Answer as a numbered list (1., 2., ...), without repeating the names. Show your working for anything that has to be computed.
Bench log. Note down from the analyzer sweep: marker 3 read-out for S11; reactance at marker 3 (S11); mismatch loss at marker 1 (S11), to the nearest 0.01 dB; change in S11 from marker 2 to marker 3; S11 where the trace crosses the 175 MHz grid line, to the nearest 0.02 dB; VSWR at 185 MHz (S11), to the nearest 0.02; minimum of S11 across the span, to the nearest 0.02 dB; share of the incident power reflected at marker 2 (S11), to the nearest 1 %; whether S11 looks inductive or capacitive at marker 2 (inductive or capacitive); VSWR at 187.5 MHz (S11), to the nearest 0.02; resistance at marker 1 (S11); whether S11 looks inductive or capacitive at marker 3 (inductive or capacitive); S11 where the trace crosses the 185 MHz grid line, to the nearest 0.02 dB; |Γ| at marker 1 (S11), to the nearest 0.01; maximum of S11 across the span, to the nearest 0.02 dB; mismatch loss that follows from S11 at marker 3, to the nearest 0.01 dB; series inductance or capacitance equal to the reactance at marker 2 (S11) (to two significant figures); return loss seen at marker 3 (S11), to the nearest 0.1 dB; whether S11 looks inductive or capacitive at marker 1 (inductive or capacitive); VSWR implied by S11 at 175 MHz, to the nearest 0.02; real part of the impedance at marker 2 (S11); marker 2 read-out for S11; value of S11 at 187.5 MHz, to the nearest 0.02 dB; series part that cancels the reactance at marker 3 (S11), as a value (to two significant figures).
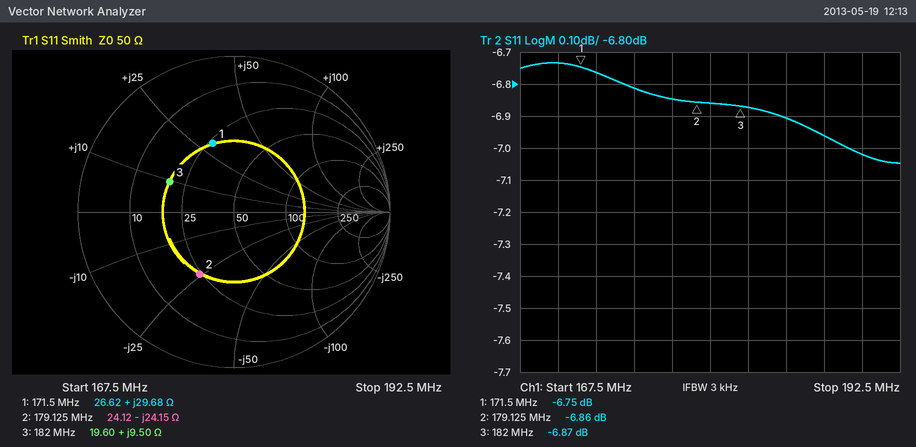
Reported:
1. -6.87 dB
2. +9.50 Ω
3. −10 log10(1 − 10^(-6.75/10)) ≈ 1.03 dB
4. -6.87 − (-6.86) = -0.01 dB
5. -6.82 dB
6. |Γ| = 10^(-6.9/20) = 0.4519; VSWR = (1 + 0.4519)/(1 − 0.4519) ≈ 2.65, so 2.64 to the nearest 0.02
7. -7.04 dB
8. 10^(-6.86/10) ≈ 21 %
9. capacitive
10. |Γ| = 10^(-6.96/20) = 0.4487; VSWR = (1 + 0.4487)/(1 − 0.4487) ≈ 2.63, so 2.62 to the nearest 0.02
11. 26.62 Ω
12. inductive
13. -6.90 dB
14. 0.46
15. -6.74 dB
16. −10 log10(1 − 10^(-6.87/10)) ≈ 1.00 dB
17. C = 1/(2π × 179.125 MHz × 24.15 Ω) ≈ 37 pF
18. 6.9 dB
19. inductive
20. |Γ| = 10^(-6.82/20) = 0.4560; VSWR = (1 + 0.4560)/(1 − 0.4560) ≈ 2.68
21. 24.12 Ω
22. -6.86 dB
23. -6.96 dB
24. C = 1/(2π × 182 MHz × 9.5 Ω) ≈ 92 pF
